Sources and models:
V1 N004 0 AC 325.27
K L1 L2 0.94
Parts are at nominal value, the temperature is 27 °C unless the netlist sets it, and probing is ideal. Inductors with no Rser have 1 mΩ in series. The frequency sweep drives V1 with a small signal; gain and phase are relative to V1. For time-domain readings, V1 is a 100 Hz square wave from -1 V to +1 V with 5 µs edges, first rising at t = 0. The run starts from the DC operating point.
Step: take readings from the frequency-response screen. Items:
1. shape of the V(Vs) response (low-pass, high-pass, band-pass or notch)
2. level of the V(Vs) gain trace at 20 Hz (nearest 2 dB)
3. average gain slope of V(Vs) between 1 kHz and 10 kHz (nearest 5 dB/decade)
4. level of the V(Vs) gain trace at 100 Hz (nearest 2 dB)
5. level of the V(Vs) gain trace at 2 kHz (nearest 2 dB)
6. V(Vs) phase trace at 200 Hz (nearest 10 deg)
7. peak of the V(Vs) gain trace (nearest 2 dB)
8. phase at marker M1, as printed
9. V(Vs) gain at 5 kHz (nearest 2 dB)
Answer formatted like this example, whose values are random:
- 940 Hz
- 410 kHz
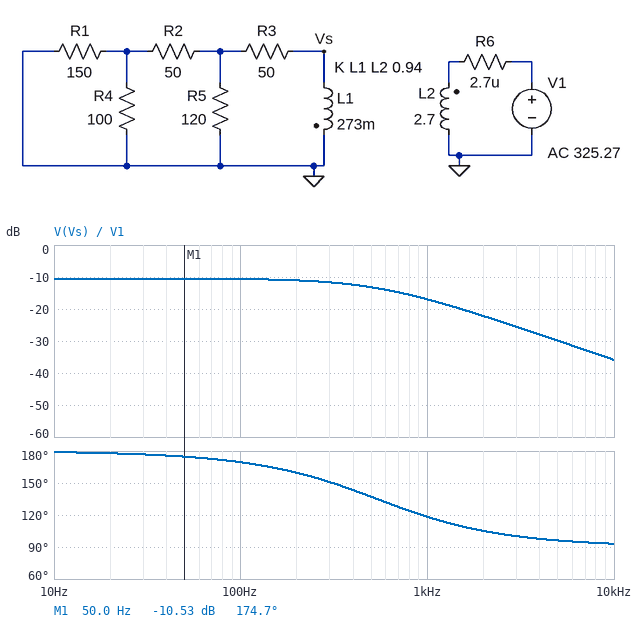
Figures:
- low-pass
- -10 dB
- -20 dB/decade
- -10 dB
- -22 dB
- 160 deg
- -10 dB
- 174.7 deg
- -30 dB
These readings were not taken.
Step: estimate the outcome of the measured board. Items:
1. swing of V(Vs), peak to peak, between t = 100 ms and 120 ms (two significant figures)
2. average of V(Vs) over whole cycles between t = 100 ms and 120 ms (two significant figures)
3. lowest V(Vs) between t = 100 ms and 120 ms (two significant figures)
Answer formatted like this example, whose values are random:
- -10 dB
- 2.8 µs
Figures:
- 600 mV
- -300 mV
- -600 mV
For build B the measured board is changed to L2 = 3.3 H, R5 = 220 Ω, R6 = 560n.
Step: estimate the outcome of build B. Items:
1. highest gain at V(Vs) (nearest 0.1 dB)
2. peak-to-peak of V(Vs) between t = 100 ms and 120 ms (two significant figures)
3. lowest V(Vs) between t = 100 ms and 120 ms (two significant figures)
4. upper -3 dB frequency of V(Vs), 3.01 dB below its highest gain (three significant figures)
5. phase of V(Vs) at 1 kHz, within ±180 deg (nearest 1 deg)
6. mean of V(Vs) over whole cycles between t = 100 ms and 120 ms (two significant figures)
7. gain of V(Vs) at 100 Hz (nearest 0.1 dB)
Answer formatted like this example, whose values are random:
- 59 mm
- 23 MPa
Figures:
- -11.4 dB
- 540 mV
- -540 mV
- 618 Hz
- 122 deg
- -270 mV
- -11.5 dB
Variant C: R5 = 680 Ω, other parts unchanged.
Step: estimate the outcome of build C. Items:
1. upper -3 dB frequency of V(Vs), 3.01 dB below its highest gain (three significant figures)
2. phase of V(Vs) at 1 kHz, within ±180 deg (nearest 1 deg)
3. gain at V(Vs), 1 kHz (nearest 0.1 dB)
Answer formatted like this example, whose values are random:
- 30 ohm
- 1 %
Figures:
- 725 Hz
- 126 deg
- -15.1 dB
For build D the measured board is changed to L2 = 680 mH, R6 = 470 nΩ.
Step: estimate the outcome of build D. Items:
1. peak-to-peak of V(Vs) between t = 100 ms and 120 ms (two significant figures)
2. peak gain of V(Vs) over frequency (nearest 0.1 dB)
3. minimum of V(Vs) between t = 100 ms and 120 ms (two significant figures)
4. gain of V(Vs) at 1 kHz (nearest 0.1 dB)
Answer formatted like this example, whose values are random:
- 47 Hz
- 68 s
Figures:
- 1.2 V
- -4.5 dB
- -1.2 V
- -11.0 dB
